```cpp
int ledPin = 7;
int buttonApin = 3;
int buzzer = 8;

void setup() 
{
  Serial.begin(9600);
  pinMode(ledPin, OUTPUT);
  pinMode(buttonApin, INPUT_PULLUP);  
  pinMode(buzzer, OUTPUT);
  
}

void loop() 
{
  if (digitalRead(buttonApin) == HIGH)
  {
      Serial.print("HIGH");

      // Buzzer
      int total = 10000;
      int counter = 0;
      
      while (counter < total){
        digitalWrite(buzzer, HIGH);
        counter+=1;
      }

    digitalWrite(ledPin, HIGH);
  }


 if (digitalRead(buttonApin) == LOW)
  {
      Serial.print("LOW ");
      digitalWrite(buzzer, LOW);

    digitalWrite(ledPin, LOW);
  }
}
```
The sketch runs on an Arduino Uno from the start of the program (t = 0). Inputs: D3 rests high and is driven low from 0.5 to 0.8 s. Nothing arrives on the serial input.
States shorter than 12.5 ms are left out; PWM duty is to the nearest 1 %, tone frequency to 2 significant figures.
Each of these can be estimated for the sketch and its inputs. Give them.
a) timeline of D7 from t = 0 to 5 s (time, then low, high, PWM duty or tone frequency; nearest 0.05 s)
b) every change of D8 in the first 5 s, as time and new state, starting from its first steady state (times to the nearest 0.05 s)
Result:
0 s low; 0.05 s high; 0.55 s low; 0.85 s high
0 s high; 0.55 s low; 0.8 s high
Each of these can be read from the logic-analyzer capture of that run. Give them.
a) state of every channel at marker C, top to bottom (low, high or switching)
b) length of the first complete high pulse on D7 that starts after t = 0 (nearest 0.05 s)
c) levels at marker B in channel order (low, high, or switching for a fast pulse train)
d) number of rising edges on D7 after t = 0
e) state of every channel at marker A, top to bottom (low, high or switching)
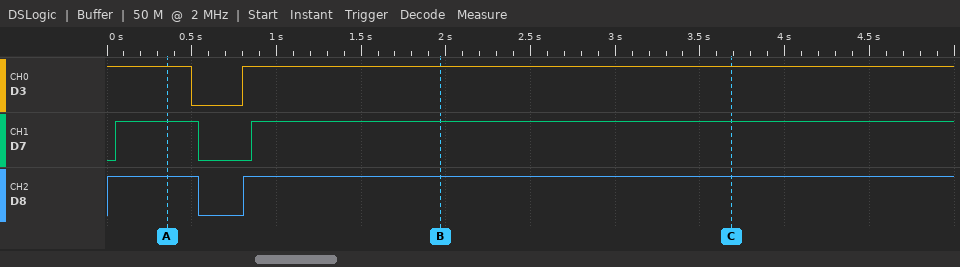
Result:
D3 high, D7 high, D8 high
0.50 s
D3 high, D7 high, D8 high
2
D3 high, D7 high, D8 high
